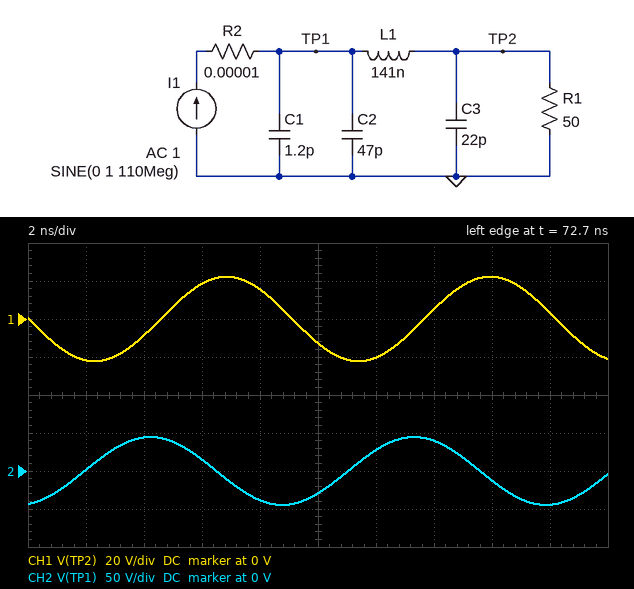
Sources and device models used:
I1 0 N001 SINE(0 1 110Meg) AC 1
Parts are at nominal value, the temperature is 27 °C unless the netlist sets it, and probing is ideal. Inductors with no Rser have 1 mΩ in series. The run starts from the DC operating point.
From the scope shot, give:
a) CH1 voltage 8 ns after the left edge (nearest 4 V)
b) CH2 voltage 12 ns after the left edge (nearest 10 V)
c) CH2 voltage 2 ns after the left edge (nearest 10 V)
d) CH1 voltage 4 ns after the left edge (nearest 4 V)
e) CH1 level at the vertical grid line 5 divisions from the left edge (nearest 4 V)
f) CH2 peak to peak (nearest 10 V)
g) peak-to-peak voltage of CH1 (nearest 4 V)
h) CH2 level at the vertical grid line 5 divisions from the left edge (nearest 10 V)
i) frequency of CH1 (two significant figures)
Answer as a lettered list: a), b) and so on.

a) 16 V
b) 30 V
c) 0 V
d) -8 V
e) -12 V
f) 90 V
g) 44 V
h) -30 V
i) 110 MHz
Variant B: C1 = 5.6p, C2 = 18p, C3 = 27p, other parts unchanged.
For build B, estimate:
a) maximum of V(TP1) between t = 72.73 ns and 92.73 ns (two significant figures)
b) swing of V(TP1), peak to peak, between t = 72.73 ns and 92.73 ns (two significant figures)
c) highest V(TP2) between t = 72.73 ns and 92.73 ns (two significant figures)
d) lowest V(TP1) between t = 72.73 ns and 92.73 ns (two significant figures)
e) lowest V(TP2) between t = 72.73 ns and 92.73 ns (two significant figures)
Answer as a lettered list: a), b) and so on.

a) 160 V
b) 330 V
c) 77 V
d) -160 V
e) -77 V
